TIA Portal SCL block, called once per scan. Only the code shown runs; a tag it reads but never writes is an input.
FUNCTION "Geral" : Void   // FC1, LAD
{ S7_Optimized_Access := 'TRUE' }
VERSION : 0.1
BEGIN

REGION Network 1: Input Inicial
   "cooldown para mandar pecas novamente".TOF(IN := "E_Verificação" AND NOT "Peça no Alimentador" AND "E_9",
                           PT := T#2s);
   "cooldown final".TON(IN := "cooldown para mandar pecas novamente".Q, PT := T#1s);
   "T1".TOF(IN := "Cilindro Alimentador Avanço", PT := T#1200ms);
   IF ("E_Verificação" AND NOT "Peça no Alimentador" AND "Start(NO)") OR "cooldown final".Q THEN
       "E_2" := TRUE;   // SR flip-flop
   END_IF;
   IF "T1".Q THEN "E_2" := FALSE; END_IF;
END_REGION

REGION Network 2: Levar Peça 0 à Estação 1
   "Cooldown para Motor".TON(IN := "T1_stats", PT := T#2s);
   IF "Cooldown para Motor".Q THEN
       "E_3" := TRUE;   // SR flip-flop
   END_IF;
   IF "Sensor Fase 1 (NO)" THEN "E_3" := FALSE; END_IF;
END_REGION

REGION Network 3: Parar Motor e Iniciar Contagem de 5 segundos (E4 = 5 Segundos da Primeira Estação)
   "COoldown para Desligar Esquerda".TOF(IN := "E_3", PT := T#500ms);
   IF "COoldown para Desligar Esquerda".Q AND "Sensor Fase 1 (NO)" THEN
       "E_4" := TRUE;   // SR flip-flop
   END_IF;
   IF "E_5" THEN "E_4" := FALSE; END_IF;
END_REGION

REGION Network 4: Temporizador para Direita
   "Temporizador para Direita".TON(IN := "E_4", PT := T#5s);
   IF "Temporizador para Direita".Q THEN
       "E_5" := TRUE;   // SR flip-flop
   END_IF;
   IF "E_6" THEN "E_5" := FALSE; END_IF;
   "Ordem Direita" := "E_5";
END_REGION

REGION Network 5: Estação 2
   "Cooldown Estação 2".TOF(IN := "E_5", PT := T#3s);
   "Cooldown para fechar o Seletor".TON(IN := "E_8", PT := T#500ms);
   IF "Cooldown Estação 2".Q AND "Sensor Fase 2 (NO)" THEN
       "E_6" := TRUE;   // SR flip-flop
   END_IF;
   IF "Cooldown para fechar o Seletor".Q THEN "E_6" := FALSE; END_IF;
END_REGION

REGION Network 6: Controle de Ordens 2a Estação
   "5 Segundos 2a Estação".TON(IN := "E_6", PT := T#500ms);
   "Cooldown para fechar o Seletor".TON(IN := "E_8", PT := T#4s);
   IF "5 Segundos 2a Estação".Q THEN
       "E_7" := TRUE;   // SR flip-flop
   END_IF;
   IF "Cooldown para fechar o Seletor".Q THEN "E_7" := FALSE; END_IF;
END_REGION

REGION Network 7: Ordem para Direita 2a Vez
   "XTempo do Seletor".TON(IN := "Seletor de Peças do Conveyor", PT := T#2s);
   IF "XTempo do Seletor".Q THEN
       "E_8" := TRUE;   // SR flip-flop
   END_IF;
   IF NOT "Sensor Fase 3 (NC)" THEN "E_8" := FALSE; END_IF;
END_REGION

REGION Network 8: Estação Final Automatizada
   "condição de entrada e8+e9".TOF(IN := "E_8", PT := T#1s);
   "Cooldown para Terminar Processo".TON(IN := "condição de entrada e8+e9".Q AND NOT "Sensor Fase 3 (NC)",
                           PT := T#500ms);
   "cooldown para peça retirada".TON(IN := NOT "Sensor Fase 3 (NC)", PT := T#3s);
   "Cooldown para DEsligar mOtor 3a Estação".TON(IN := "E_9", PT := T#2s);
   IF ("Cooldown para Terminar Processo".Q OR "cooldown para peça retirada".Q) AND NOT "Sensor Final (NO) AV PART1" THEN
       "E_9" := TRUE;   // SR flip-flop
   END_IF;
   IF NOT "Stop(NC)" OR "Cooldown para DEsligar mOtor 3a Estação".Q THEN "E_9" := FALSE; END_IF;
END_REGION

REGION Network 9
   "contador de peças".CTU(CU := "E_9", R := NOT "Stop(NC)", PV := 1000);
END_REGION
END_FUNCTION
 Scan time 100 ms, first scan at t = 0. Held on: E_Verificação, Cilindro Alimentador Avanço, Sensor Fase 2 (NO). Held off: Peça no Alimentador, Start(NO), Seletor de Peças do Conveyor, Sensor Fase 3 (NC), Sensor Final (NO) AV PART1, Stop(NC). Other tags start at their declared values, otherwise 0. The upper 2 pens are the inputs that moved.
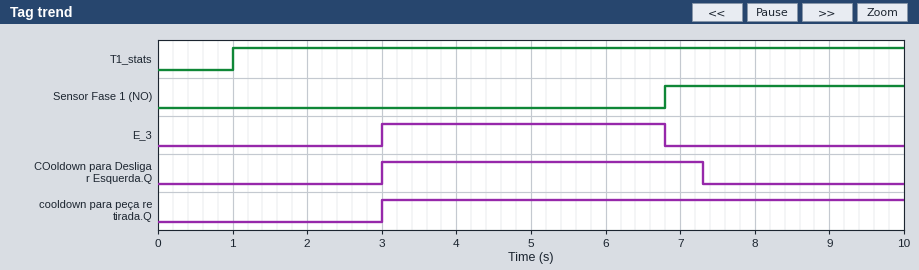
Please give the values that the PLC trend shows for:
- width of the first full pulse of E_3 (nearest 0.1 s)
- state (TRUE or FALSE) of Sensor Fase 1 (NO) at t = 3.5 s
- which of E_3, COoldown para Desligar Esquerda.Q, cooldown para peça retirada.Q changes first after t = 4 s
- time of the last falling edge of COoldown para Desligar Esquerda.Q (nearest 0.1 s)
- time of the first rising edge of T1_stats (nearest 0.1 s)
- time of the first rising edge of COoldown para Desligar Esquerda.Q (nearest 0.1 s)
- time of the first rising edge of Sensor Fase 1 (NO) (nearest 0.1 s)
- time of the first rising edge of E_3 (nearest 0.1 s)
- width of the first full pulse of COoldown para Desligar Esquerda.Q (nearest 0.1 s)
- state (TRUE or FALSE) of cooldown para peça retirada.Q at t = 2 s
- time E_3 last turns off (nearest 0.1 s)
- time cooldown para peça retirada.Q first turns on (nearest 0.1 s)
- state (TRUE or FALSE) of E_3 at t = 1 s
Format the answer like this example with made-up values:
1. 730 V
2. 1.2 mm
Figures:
1. 3.8 s
2. FALSE
3. E_3
4. 7.3 s
5. 1.0 s
6. 3.0 s
7. 6.8 s
8. 3.0 s
9. 4.3 s
10. FALSE
11. 6.8 s
12. 3.0 s
13. FALSE
